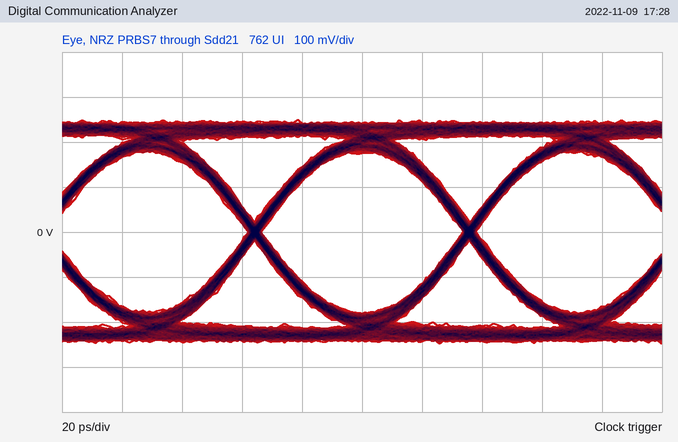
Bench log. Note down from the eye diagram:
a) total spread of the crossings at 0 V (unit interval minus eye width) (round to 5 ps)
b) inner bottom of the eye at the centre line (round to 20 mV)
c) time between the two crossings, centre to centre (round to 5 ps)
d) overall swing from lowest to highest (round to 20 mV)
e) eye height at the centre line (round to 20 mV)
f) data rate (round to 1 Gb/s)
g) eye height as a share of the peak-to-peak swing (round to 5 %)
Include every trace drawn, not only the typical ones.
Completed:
5 ps
-180 mV
70 ps
500 mV
360 mV
14 Gb/s
70 %
